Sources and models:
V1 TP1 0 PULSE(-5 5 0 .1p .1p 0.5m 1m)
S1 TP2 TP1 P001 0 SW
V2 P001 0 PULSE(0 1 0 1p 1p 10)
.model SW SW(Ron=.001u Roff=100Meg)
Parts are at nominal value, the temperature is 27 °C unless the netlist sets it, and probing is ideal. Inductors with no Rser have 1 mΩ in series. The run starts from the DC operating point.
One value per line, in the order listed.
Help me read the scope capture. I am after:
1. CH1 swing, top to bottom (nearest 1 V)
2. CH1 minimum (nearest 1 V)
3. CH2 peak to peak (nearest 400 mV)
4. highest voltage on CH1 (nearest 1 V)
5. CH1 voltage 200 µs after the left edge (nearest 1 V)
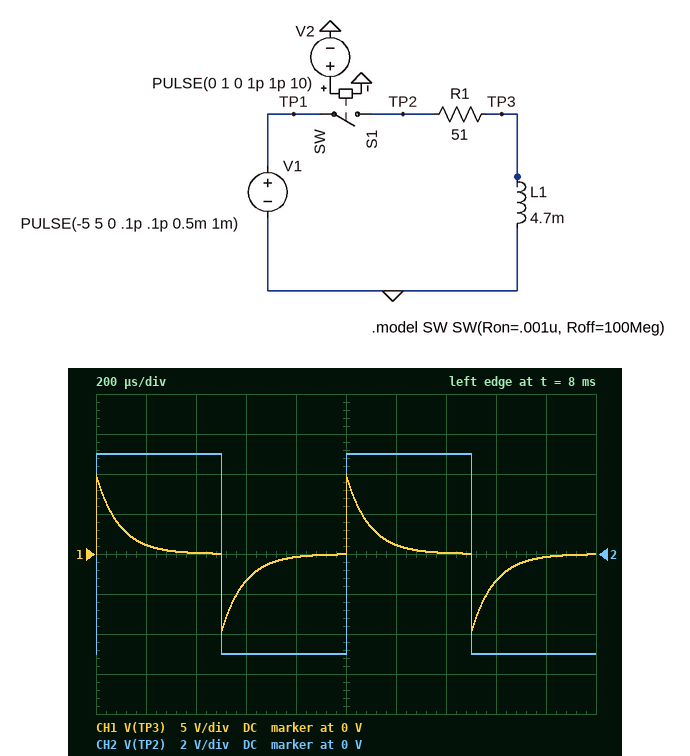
20 V
-10 V
10.0 V
10 V
1 V
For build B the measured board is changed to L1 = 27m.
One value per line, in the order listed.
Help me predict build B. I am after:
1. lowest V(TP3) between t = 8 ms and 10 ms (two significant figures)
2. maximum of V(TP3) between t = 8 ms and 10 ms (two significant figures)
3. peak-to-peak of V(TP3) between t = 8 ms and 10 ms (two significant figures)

-7.2 V
7.2 V
14 V
